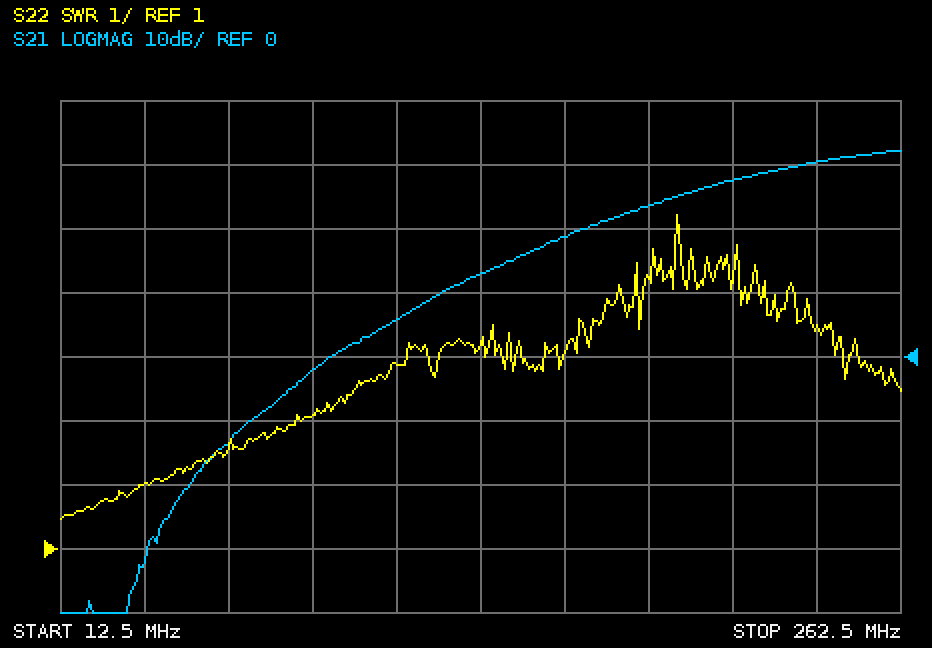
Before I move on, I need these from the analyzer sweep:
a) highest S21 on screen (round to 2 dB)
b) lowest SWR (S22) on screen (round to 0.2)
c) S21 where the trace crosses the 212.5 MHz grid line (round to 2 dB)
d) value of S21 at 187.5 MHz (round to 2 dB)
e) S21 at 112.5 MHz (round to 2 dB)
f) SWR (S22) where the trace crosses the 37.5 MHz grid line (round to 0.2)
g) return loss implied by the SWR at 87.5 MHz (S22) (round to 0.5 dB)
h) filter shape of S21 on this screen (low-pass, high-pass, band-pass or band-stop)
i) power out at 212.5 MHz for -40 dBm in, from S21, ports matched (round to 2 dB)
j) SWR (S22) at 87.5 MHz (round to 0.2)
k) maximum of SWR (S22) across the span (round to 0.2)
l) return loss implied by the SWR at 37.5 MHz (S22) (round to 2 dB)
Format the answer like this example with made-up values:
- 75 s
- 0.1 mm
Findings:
- 32 dB
- 1.4
- 28 dB
- 24 dB
- 6 dB
- 2.0
- 6.0 dB
- high-pass
- -12 dBm
- 3.0
- 6.2
- 10 dB
